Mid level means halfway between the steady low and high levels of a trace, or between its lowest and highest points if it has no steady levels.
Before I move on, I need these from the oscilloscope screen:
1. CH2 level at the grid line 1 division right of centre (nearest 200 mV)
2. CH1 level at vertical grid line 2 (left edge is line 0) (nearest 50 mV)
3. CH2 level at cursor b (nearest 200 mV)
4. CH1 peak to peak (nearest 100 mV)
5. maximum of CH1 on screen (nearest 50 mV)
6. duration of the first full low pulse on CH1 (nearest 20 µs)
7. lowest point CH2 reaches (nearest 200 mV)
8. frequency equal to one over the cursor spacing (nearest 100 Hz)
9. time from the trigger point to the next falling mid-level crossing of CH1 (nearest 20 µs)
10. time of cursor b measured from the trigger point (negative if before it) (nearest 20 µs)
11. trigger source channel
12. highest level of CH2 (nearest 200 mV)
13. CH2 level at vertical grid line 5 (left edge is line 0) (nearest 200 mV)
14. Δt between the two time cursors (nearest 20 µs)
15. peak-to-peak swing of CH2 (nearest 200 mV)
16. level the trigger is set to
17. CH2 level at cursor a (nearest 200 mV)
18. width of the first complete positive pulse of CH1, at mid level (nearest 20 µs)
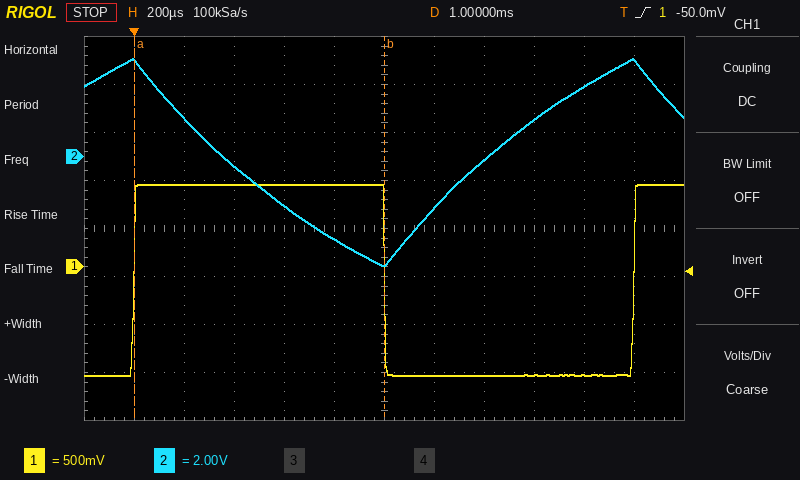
-2.2 V
850 mV
-4.4 V
2.00 V
850 mV
1.00 ms
-4.6 V
1.0 kHz
1.00 ms
+1.00 ms
CH1
4.0 V
-3.4 V
1.00 ms
8.6 V
-50.0 mV
4.0 V
1.00 ms
